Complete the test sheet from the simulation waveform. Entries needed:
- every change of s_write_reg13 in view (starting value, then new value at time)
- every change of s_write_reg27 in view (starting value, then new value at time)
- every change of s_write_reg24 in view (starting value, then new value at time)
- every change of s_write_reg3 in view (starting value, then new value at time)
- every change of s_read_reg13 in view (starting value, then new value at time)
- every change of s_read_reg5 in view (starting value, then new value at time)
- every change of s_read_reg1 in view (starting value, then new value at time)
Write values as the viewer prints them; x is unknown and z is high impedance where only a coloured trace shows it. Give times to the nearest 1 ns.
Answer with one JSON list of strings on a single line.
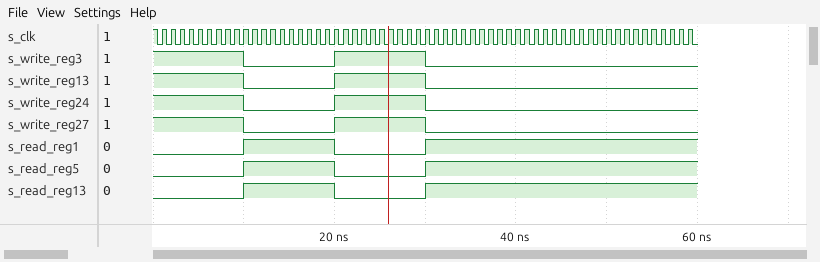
["1, 0 at 10 ns, 1 at 20 ns, 0 at 30 ns", "1, 0 at 10 ns, 1 at 20 ns, 0 at 30 ns", "1, 0 at 10 ns, 1 at 20 ns, 0 at 30 ns", "1, 0 at 10 ns, 1 at 20 ns, 0 at 30 ns", "0, 1 at 10 ns, 0 at 20 ns, 1 at 30 ns", "0, 1 at 10 ns, 0 at 20 ns, 1 at 30 ns", "0, 1 at 10 ns, 0 at 20 ns, 1 at 30 ns"]
